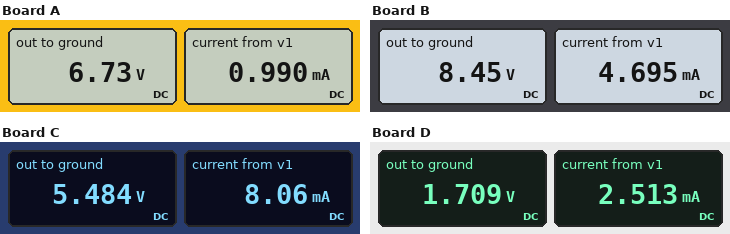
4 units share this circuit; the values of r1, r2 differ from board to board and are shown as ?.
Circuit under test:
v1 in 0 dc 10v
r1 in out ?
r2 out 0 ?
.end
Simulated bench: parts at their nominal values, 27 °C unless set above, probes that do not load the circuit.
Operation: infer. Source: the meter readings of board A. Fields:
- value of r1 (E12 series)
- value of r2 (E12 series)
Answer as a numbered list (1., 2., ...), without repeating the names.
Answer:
1. 3.3 kΩ
2. 6.8 kΩ
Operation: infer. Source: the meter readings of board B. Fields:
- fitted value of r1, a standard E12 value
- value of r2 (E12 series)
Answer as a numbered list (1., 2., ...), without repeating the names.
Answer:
1. 330 Ω
2. 1.8 kΩ
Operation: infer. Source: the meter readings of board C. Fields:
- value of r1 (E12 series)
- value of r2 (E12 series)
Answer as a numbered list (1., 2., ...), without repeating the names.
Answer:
1. 560 Ω
2. 680 Ω
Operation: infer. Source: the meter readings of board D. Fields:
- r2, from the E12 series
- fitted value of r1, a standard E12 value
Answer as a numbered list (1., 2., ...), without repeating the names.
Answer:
1. 680 Ω
2. 3.3 kΩ
